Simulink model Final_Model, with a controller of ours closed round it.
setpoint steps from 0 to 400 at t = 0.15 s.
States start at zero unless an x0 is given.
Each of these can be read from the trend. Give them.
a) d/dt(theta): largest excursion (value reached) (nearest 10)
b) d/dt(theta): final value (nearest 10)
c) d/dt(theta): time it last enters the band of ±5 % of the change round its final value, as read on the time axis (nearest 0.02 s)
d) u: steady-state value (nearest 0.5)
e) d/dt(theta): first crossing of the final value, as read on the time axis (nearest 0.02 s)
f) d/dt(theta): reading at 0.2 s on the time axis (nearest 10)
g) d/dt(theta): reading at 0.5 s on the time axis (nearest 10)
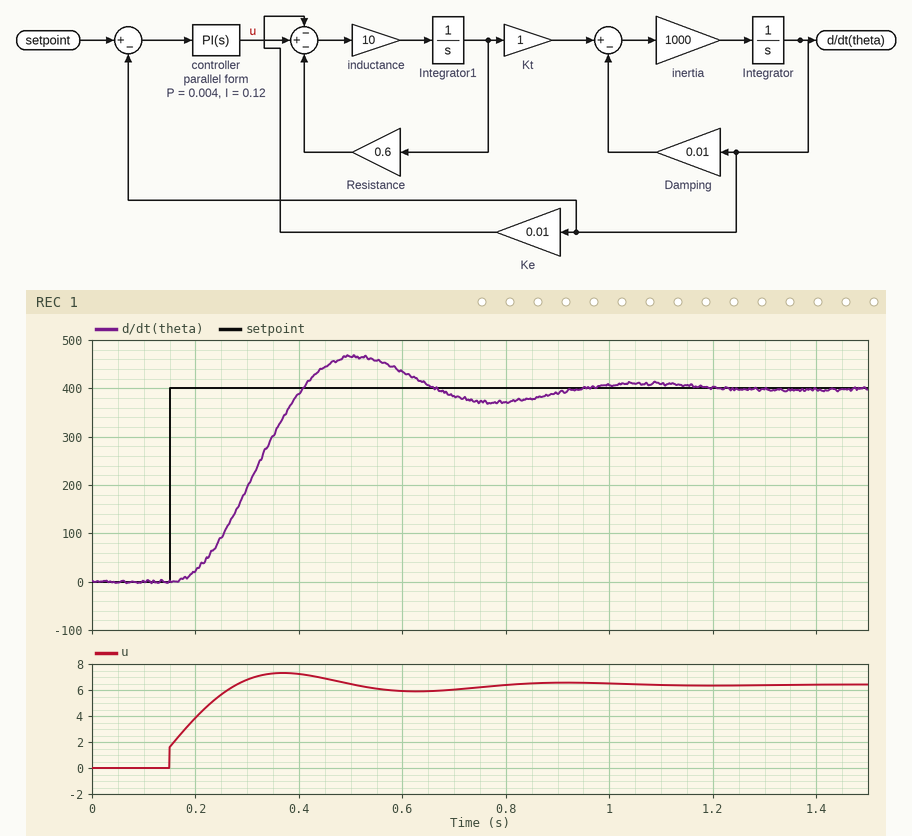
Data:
470
400
0.86 s
6.5
0.40 s
20
470
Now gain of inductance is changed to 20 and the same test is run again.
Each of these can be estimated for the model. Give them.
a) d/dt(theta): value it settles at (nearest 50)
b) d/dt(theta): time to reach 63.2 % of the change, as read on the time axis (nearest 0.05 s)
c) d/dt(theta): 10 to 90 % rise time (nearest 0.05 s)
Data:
400
0.30 s
0.15 s
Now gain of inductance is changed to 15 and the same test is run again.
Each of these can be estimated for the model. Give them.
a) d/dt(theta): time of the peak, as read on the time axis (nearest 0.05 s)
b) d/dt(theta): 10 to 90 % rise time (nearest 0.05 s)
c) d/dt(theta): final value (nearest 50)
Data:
0.45 s
0.15 s
400
